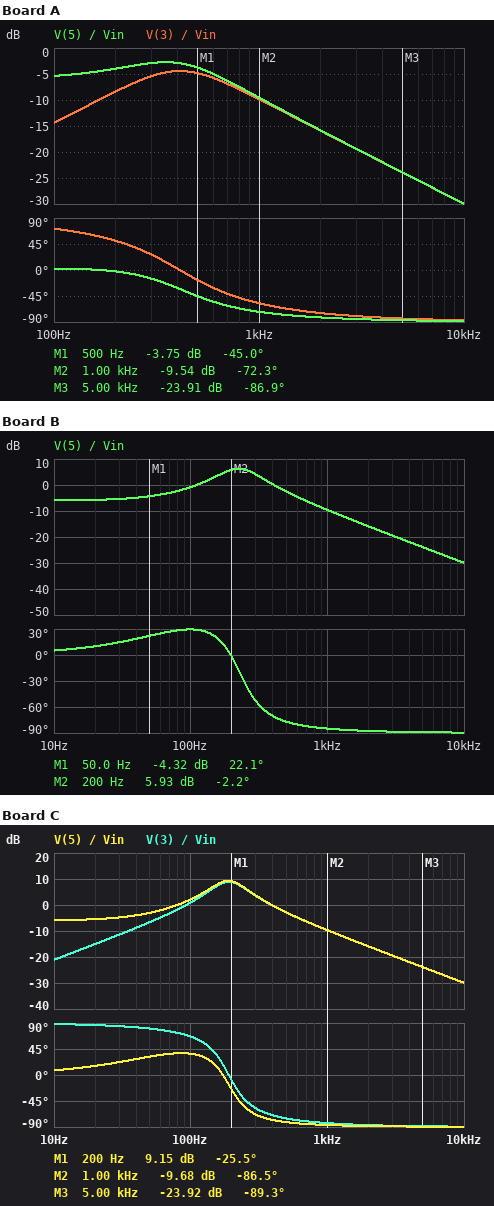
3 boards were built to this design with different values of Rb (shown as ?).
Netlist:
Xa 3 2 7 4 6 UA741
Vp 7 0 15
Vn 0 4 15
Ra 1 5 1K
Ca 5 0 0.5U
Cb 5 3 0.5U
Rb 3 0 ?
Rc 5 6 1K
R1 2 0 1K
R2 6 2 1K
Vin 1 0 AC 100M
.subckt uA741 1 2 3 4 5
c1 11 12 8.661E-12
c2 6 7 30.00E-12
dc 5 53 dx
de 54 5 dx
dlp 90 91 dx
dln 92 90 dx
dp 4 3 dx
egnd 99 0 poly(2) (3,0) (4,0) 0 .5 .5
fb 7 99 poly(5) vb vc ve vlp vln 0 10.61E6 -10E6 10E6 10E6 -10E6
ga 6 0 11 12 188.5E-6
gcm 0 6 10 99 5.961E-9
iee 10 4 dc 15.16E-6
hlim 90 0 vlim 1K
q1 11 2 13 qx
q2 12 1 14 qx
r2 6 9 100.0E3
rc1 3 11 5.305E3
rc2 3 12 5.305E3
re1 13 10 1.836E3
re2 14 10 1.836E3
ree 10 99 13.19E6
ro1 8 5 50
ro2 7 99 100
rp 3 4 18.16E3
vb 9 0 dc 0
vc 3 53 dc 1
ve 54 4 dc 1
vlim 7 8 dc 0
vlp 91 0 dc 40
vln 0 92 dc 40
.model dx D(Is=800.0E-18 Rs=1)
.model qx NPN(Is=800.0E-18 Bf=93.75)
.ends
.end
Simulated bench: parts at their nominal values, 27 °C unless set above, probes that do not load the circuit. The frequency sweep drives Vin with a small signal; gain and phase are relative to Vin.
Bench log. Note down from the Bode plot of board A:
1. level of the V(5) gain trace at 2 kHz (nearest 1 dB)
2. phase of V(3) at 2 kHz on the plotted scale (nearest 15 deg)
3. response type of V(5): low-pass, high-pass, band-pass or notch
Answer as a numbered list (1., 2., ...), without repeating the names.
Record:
1. -16 dB
2. -75 deg
3. low-pass
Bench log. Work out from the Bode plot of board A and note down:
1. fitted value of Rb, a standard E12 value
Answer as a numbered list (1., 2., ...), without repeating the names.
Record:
1. 1.2 kΩ
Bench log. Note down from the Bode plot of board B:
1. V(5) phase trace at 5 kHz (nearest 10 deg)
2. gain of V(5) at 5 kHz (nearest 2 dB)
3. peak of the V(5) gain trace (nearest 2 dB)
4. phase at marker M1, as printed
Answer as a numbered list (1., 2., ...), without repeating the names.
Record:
1. -90 deg
2. -24 dB
3. 6 dB
4. 22.1 deg
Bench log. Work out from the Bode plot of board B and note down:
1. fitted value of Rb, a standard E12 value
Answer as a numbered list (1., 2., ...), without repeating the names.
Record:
1. 3.9 kΩ
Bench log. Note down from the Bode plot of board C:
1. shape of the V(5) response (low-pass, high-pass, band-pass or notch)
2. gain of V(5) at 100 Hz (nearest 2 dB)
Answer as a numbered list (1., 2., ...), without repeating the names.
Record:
1. band-pass
2. 2 dB
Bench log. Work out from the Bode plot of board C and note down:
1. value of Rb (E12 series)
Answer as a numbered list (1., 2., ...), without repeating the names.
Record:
1. 5.6 kΩ
